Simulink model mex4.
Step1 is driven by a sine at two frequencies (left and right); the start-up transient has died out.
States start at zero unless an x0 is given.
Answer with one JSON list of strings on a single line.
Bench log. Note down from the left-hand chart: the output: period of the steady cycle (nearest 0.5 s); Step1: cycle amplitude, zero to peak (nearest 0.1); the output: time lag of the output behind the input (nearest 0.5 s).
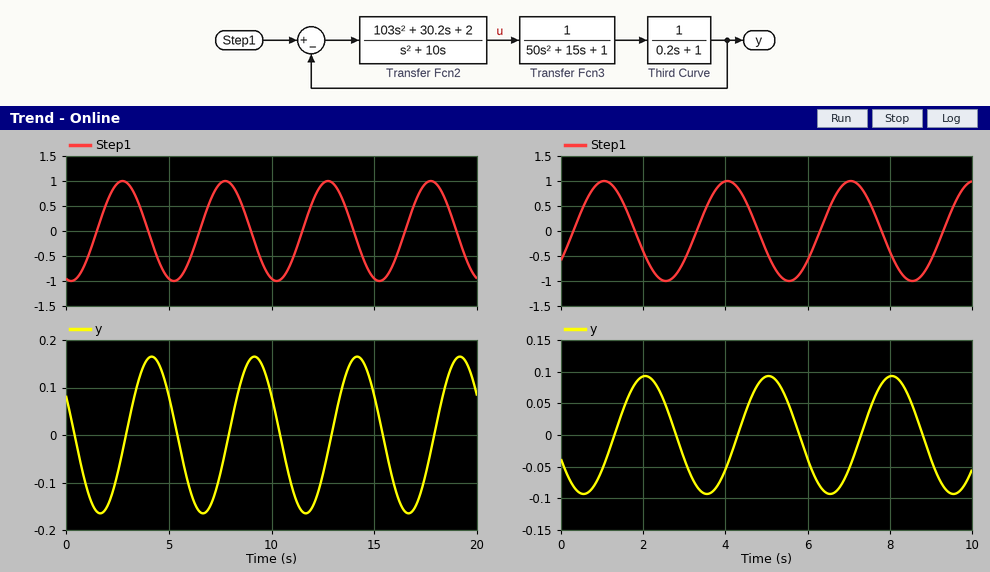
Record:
["5.0 s", "1.0", "1.5 s"]
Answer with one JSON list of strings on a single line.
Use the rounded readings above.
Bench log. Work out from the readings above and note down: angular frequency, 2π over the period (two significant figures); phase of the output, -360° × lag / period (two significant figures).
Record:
["1.3 rad/s", "-110°"]
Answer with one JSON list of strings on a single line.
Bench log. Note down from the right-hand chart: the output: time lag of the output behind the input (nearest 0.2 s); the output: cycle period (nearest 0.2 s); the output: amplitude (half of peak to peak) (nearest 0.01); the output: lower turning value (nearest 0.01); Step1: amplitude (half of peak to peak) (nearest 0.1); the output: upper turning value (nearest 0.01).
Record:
["1.0 s", "3.0 s", "0.09", "-0.09", "1.0", "0.09"]
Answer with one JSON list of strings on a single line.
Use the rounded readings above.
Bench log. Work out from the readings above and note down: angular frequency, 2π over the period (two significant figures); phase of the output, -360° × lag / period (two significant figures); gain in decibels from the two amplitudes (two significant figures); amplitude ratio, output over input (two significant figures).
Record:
["2.1 rad/s", "-120°", "-21 dB", "0.090"]
